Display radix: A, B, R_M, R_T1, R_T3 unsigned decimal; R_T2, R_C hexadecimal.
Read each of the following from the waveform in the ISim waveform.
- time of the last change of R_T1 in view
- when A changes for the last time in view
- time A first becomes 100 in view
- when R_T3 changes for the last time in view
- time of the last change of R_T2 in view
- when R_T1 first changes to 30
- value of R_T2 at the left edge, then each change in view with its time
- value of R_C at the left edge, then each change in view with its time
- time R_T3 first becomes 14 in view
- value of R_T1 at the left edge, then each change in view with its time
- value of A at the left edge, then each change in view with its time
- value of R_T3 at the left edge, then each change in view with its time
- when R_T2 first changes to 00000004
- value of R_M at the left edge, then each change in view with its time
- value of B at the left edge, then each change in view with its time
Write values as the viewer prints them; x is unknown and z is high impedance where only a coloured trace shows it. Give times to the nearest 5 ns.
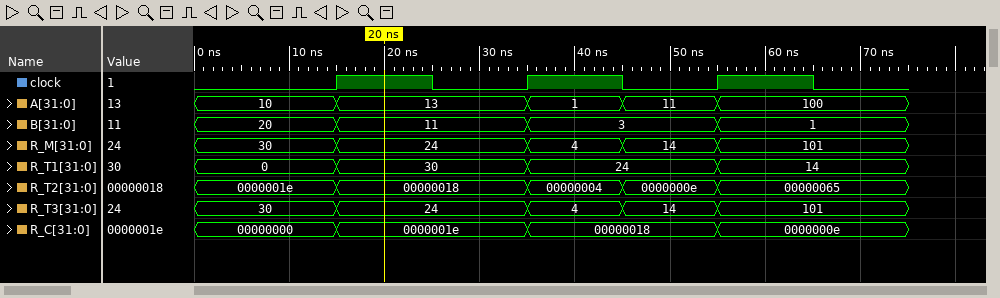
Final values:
55 ns
55 ns
55 ns
55 ns
55 ns
15 ns
0000001e, 00000018 at 15 ns, 00000004 at 35 ns, 0000000e at 45 ns, 00000065 at 55 ns
00000000, 0000001e at 15 ns, 00000018 at 35 ns, 0000000e at 55 ns
45 ns
0, 30 at 15 ns, 24 at 35 ns, 14 at 55 ns
10, 13 at 15 ns, 1 at 35 ns, 11 at 45 ns, 100 at 55 ns
30, 24 at 15 ns, 4 at 35 ns, 14 at 45 ns, 101 at 55 ns
35 ns
30, 24 at 15 ns, 4 at 35 ns, 14 at 45 ns, 101 at 55 ns
20, 11 at 15 ns, 3 at 35 ns, 1 at 55 ns
